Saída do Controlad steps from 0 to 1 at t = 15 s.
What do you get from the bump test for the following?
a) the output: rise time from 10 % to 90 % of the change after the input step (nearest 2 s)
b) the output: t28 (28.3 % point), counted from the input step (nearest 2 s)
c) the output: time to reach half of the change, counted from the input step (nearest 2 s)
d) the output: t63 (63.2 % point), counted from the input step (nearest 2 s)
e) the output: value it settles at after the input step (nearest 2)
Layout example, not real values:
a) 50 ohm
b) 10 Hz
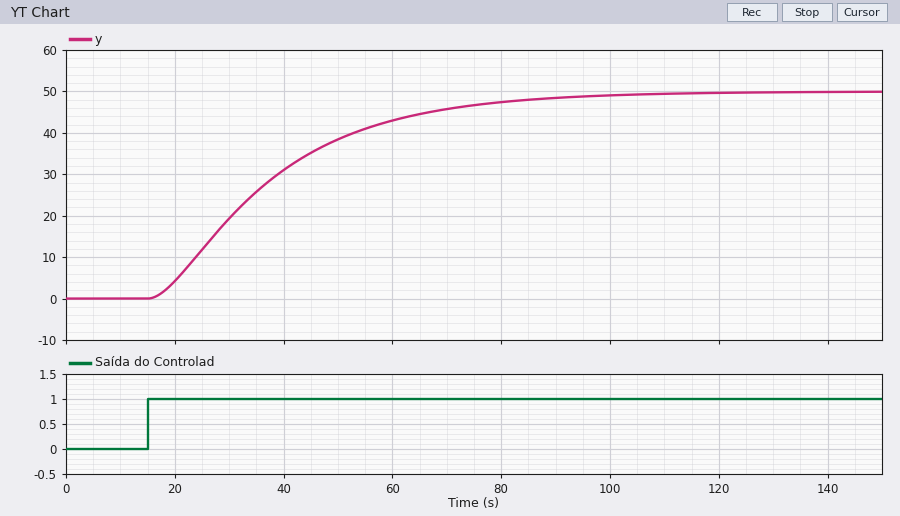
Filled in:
a) 46 s
b) 12 s
c) 20 s
d) 26 s
e) 50
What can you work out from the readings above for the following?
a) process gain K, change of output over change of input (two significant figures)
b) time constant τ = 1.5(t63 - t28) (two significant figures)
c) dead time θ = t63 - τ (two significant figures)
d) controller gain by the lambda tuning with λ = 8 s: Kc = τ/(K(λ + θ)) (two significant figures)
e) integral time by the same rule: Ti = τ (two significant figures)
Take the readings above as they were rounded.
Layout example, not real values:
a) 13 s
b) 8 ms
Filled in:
a) 50
b) 21 s
c) 5.0 s
d) 0.032
e) 21 s
